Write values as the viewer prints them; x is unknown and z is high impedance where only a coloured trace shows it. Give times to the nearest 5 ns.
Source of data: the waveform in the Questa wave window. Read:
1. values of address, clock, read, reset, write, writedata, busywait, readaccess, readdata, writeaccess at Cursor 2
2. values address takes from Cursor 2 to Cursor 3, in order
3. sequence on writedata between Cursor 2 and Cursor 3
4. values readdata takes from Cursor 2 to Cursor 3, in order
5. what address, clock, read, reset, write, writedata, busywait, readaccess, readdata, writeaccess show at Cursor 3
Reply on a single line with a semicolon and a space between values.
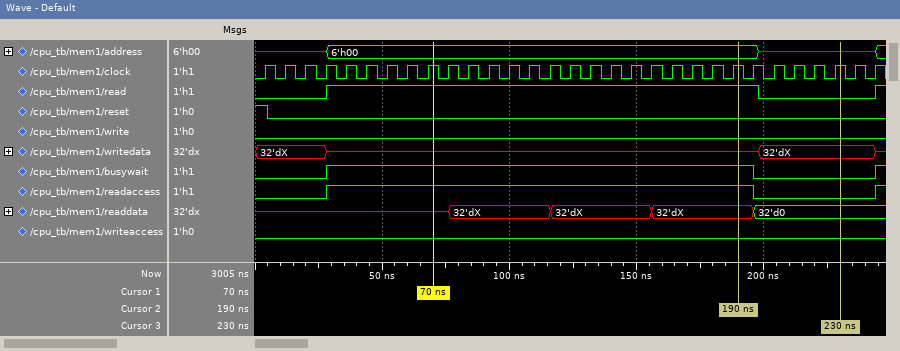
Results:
address=6'h00, clock=1, read=1, reset=0, write=0, writedata=x, busywait=1, readaccess=1, readdata=32'dX, writeaccess=0; 6'h00, x; x, 32'dX; 32'dX, 32'd0; address=x, clock=1, read=0, reset=0, write=0, writedata=32'dX, busywait=0, readaccess=0, readdata=32'd0, writeaccess=0
